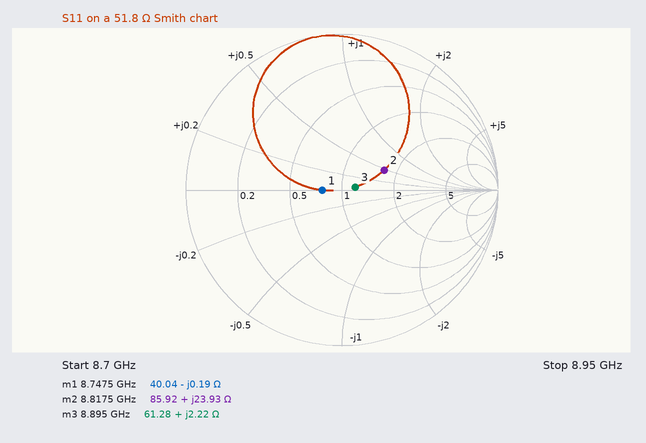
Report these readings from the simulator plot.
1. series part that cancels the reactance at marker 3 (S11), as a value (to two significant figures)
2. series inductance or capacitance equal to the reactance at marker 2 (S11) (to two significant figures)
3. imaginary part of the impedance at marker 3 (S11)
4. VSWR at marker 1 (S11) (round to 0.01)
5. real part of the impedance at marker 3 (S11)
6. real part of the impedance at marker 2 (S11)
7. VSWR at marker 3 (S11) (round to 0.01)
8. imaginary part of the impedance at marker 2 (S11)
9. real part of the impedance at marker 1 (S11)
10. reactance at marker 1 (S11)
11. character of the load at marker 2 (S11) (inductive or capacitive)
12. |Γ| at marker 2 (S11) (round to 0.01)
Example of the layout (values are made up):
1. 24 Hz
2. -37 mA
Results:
1. 8.1 pF
2. 430 pH
3. +2.22 Ω
4. 1.29
5. 61.28 Ω
6. 85.92 Ω
7. 1.19
8. +23.93 Ω
9. 40.04 Ω
10. -0.19 Ω
11. inductive
12. 0.30
